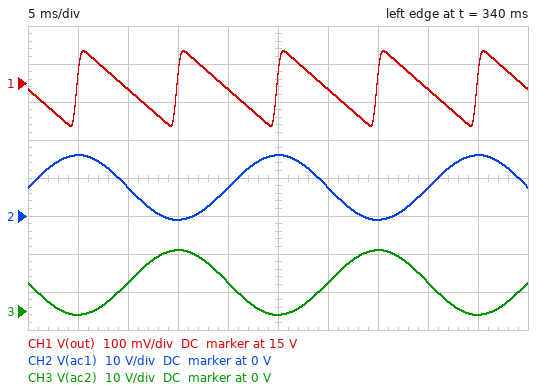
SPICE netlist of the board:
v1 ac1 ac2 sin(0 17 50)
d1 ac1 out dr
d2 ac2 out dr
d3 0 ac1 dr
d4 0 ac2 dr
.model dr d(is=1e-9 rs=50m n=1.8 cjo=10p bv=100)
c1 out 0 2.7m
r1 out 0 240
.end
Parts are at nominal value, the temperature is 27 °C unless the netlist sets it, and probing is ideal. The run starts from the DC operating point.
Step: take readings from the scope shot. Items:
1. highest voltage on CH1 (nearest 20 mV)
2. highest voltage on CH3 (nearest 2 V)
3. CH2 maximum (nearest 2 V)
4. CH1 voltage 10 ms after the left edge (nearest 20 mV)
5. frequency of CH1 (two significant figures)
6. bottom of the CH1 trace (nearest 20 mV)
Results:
15.08 V
16 V
16 V
14.98 V
100 Hz
14.88 V
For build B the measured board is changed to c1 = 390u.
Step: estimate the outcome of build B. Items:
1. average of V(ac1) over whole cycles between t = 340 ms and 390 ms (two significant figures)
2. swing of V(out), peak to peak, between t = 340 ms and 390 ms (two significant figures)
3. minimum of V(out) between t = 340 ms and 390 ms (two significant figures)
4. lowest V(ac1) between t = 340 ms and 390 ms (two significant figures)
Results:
7.3 V
1.3 V
14 V
-980 mV
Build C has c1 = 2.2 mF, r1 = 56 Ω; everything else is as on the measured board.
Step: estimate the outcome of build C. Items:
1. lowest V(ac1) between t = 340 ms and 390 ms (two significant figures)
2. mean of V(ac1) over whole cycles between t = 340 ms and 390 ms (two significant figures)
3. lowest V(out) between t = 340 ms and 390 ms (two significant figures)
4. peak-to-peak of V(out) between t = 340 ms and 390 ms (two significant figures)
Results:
-1.1 V
7.3 V
14 V
970 mV
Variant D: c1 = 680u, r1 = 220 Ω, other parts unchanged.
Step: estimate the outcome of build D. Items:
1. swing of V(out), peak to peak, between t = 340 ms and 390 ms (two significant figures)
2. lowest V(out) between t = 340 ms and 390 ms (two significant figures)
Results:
830 mV
14 V
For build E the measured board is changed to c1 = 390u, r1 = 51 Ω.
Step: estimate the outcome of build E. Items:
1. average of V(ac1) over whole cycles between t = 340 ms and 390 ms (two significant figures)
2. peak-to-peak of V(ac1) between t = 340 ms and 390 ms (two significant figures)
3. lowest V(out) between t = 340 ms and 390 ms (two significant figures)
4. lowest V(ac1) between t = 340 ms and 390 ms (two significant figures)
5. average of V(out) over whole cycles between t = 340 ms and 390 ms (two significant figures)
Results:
6.5 V
17 V
11 V
-1.1 V
13 V
